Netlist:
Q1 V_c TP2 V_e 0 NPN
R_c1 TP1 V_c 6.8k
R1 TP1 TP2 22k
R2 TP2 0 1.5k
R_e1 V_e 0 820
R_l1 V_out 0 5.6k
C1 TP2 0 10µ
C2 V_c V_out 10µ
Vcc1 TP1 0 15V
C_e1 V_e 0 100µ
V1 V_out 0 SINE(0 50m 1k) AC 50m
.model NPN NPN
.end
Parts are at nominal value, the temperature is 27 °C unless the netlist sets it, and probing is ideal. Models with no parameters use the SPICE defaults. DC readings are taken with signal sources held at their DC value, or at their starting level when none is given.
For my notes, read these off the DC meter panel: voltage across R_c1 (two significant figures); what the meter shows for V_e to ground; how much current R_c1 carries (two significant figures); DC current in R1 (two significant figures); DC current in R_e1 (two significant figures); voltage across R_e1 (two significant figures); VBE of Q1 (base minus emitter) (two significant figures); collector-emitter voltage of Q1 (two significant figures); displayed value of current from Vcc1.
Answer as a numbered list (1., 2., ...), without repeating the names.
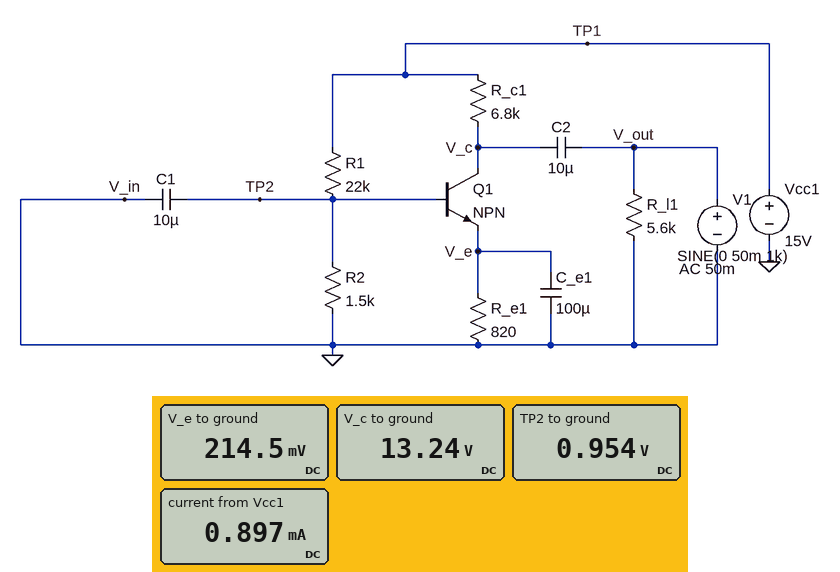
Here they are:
1. 1.8 V
2. 214.5 mV
3. 260 µA
4. 640 µA
5. 260 µA
6. 210 mV
7. 740 mV
8. 13 V
9. 0.897 mA
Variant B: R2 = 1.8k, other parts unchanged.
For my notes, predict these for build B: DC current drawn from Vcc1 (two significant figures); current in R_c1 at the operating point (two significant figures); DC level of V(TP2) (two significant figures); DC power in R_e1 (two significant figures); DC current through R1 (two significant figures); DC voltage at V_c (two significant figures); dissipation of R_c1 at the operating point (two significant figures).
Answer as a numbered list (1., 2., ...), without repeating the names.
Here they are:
1. 1.1 mA
2. 450 µA
3. 1.1 V
4. 170 µW
5. 630 µA
6. 12 V
7. 1.4 mW
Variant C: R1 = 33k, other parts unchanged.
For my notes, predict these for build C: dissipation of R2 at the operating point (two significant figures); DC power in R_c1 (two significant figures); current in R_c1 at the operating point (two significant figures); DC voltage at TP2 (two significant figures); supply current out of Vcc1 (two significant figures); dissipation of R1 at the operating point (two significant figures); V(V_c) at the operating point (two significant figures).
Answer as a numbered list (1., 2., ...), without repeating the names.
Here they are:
1. 280 µW
2. 340 nW
3. 7.1 µA
4. 650 mV
5. 440 µA
6. 6.2 mW
7. 15 V
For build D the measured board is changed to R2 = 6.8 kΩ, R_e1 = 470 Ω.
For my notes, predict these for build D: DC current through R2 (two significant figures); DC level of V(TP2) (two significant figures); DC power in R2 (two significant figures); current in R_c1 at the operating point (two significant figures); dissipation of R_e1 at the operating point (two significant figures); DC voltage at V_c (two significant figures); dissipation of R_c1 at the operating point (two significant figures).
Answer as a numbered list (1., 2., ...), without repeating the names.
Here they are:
1. 280 µA
2. 1.9 V
3. 530 µW
4. 2.0 mA
5. 2.6 mW
6. 1.2 V
7. 28 mW
